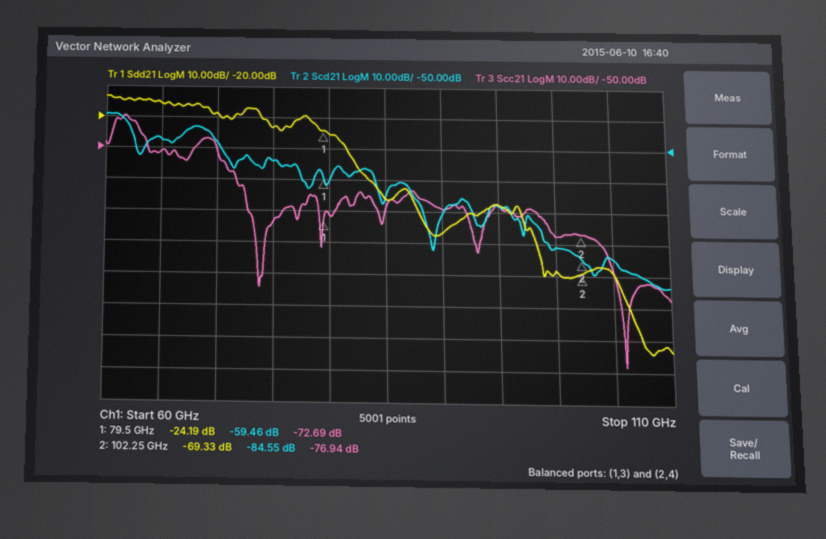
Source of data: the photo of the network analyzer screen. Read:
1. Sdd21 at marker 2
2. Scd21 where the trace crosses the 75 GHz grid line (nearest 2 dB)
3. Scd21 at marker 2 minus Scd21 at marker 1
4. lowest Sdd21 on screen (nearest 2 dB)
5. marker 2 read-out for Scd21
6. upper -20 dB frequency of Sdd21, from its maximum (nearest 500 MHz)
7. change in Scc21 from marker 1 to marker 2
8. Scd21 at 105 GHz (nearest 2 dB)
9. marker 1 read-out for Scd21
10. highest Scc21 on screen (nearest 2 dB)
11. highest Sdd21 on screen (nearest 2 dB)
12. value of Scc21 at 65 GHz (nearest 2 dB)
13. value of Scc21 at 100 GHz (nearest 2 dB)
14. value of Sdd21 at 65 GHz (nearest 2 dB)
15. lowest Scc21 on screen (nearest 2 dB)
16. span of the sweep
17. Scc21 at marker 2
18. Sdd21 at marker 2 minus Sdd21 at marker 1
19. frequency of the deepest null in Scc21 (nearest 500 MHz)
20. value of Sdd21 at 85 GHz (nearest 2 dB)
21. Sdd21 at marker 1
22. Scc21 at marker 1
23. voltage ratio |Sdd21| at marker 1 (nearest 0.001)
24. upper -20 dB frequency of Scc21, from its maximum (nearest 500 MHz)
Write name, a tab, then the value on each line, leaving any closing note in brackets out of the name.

Sdd21 at marker 2	-69.33 dB
Scd21 where the trace crosses the 75 GHz grid line	-54 dB
Scd21 at marker 2 minus Scd21 at marker 1	-25.09 dB
lowest Sdd21 on screen	-94 dB
marker 2 read-out for Scd21	-84.55 dB
upper -20 dB frequency of Sdd21, from its maximum	82.0 GHz
change in Scc21 from marker 1 to marker 2	-4.25 dB
Scd21 at 105 GHz	-84 dB
marker 1 read-out for Scd21	-59.46 dB
highest Scc21 on screen	-40 dB
highest Sdd21 on screen	-14 dB
value of Scc21 at 65 GHz	-52 dB
value of Scc21 at 100 GHz	-78 dB
value of Sdd21 at 65 GHz	-16 dB
lowest Scc21 on screen	-118 dB
span of the sweep	50 GHz
Scc21 at marker 2	-76.94 dB
Sdd21 at marker 2 minus Sdd21 at marker 1	-45.14 dB
frequency of the deepest null in Scc21	106.0 GHz
value of Sdd21 at 85 GHz	-46 dB
Sdd21 at marker 1	-24.19 dB
Scc21 at marker 1	-72.69 dB
voltage ratio |Sdd21| at marker 1	0.062
upper -20 dB frequency of Scc21, from its maximum	71.5 GHz
